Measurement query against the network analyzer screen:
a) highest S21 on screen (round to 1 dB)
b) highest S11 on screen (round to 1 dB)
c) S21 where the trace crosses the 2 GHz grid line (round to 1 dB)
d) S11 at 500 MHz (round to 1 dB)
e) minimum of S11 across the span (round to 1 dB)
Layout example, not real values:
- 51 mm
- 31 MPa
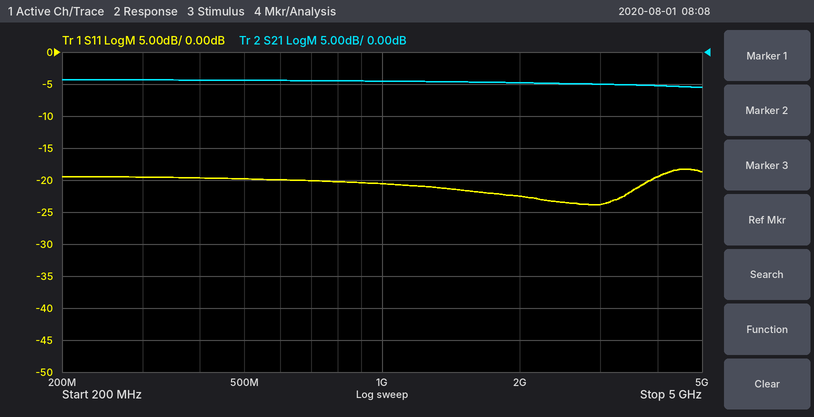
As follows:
- -4 dB
- -18 dB
- -5 dB
- -20 dB
- -24 dB
